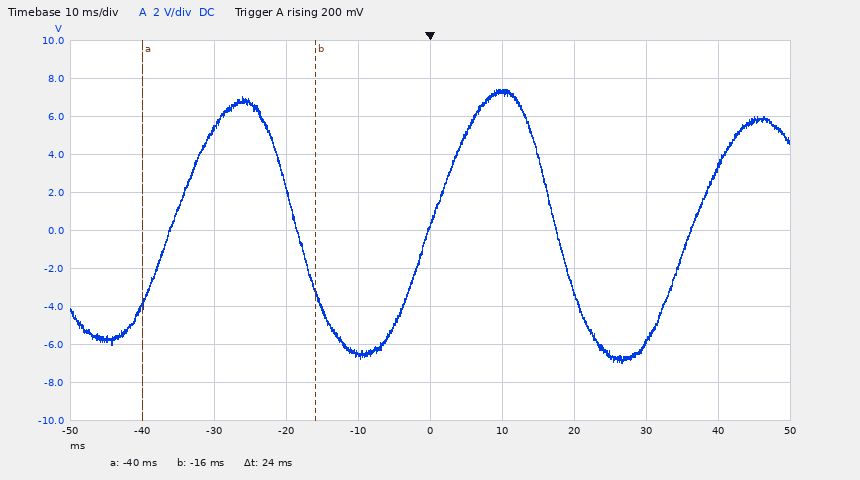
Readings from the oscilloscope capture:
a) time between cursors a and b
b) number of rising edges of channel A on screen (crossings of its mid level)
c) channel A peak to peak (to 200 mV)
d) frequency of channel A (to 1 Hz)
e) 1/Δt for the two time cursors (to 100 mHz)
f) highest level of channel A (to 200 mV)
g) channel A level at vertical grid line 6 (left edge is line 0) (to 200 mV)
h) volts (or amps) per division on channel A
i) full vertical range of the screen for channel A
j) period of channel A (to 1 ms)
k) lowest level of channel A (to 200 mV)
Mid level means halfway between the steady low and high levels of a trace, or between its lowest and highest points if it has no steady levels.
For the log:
24 ms
3
14.4 V
28 Hz
41.7 Hz
7.4 V
7.2 V
2 V
20 V
36 ms
-7.0 V
